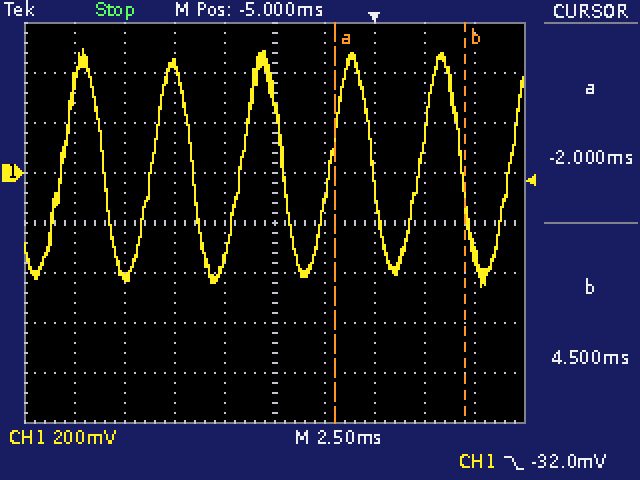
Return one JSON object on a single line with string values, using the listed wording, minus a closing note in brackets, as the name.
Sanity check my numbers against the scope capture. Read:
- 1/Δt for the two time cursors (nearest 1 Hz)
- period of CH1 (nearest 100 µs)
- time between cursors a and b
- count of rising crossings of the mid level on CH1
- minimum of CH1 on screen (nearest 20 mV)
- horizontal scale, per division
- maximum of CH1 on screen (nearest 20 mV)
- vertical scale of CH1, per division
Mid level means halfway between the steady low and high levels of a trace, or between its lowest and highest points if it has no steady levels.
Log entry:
{"1/Δt for the two time cursors": "154 Hz", "period of CH1": "4.5 ms", "time between cursors a and b": "6.50 ms", "count of rising crossings of the mid level on CH1": "6", "minimum of CH1 on screen": "-460 mV", "horizontal scale, per division": "2.5 ms", "maximum of CH1 on screen": "500 mV", "vertical scale of CH1, per division": "200 mV"}
